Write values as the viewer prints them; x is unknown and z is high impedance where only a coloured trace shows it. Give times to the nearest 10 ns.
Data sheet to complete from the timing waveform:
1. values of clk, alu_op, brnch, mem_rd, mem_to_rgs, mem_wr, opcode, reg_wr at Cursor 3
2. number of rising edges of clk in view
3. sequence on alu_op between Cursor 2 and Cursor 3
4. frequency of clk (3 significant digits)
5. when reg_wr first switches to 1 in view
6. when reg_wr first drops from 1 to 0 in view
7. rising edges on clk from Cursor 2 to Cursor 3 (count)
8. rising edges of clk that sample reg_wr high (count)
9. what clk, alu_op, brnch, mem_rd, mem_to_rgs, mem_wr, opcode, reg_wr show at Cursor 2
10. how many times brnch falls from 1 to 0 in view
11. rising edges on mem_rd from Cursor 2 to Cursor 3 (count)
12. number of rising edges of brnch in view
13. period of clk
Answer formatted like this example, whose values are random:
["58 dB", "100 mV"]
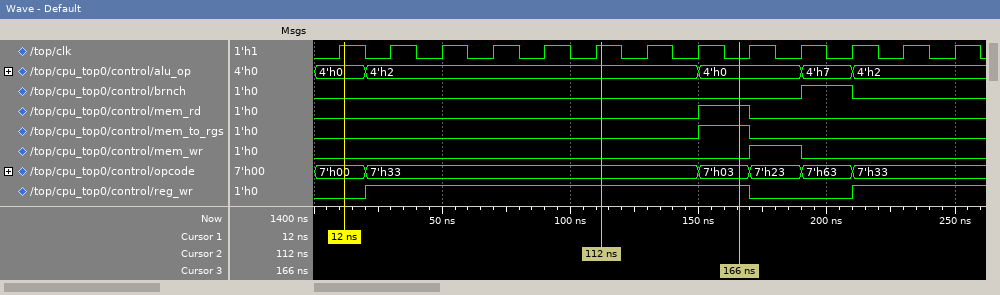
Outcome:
["clk=0, alu_op=4'h0, brnch=0, mem_rd=1, mem_to_rgs=1, mem_wr=0, opcode=7'h03, reg_wr=1", "13", "4'h2, 4'h0", "50.0 MHz", "20 ns", "170 ns", "2", "10", "clk=1, alu_op=4'h2, brnch=0, mem_rd=0, mem_to_rgs=0, mem_wr=0, opcode=7'h33, reg_wr=1", "1", "1", "1", "20 ns"]
